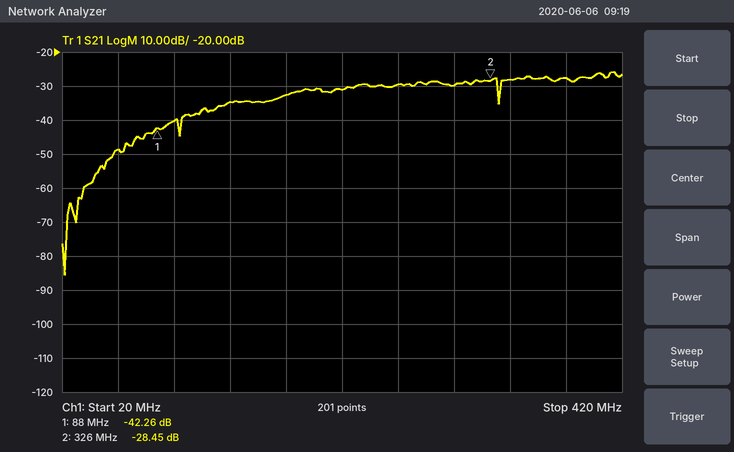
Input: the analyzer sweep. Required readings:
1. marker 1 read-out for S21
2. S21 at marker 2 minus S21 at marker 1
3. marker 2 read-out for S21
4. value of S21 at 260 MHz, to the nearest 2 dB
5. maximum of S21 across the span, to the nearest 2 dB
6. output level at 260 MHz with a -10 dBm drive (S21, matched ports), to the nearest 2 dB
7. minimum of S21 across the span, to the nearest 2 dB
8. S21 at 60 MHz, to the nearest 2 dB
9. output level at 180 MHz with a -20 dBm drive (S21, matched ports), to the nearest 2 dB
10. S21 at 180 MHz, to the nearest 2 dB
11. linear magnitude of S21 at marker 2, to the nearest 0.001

-42.26 dB
13.81 dB
-28.45 dB
-30 dB
-26 dB
-40 dBm
-86 dB
-48 dB
-52 dBm
-32 dB
0.038
